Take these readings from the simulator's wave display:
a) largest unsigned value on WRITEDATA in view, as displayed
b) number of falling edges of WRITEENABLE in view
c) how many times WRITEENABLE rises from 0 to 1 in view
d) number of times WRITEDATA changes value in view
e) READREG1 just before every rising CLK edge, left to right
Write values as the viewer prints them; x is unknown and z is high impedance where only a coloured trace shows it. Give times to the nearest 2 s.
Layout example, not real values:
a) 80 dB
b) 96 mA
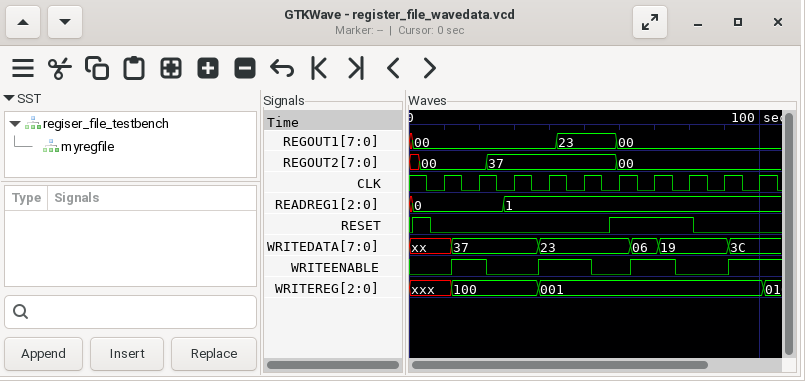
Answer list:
a) 3C
b) 3
c) 4
d) 5
e) 0, 0, 1, 1, 1, 1, 1, 1, 1, 1
